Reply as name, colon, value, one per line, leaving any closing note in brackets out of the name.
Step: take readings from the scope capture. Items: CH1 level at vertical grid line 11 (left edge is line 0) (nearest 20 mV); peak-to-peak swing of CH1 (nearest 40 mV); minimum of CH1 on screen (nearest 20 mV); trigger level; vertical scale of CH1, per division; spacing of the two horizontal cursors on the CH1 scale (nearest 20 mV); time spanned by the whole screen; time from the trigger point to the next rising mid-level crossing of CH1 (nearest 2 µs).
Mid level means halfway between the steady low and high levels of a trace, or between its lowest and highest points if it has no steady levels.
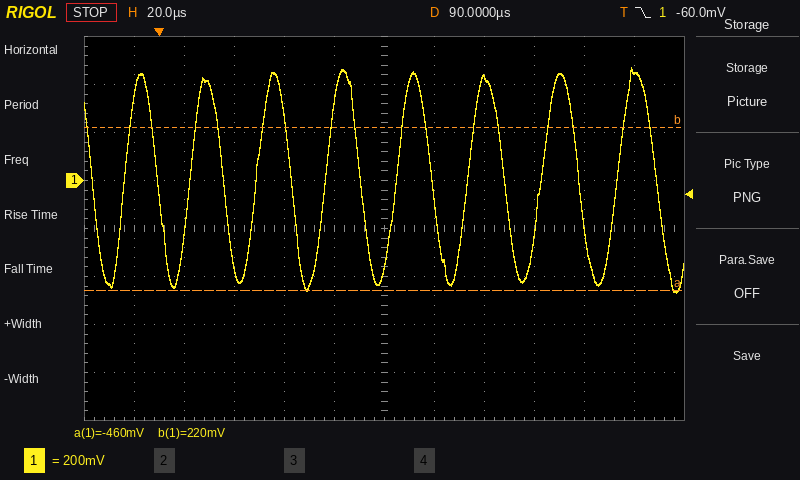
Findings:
CH1 level at vertical grid line 11 (left edge is line 0): 460 mV
peak-to-peak swing of CH1: 920 mV
minimum of CH1 on screen: -460 mV
trigger level: -60.0 mV
vertical scale of CH1, per division: 200 mV
spacing of the two horizontal cursors on the CH1 scale: 680 mV
time spanned by the whole screen: 240 µs
time from the trigger point to the next rising mid-level crossing of CH1: 12 µs
